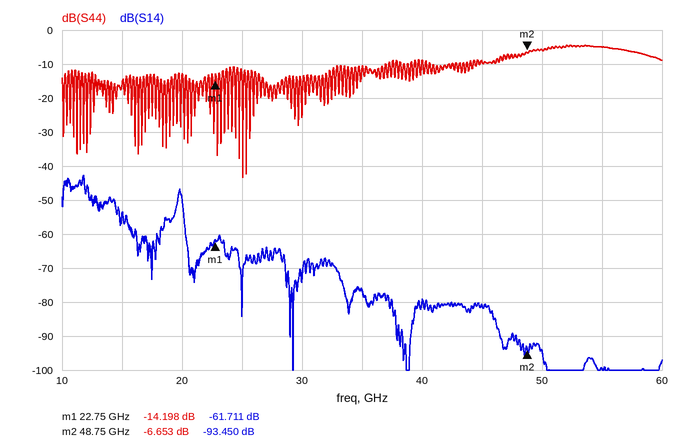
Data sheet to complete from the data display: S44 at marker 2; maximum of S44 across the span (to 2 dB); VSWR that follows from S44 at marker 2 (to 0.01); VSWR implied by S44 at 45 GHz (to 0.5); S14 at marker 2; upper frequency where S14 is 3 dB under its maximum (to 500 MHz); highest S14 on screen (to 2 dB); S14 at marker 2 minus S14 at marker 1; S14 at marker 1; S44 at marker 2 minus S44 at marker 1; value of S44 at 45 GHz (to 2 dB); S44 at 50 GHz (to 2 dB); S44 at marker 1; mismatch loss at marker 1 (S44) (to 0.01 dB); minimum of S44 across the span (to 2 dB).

-6.653 dB
-4 dB
2.74
2.0
-93.450 dB
12.0 GHz
-42 dB
-31.739 dB
-61.711 dB
7.545 dB
-10 dB
-6 dB
-14.198 dB
0.17 dB
-44 dB
